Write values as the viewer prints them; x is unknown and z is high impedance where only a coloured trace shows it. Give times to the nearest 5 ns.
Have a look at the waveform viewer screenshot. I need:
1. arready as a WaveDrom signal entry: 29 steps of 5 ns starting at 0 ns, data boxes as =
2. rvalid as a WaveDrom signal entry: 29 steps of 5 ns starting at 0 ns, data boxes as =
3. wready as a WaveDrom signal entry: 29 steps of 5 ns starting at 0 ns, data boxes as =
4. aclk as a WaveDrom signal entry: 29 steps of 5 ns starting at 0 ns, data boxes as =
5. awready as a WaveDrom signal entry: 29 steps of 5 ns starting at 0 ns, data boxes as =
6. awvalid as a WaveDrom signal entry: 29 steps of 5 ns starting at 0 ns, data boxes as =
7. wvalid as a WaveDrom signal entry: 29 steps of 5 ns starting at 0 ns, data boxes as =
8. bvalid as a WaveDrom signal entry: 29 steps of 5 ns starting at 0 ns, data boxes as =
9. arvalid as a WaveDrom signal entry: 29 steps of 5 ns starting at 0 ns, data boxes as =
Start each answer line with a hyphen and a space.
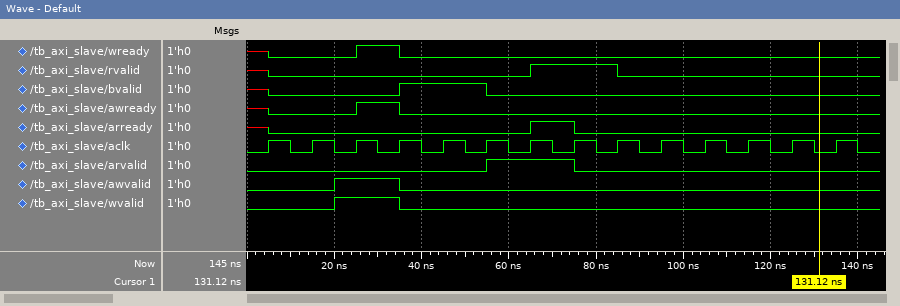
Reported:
- {name: 'arready', wave: 'x0...........1.0.............'}
- {name: 'rvalid', wave: 'x0...........1...0...........'}
- {name: 'wready', wave: 'x0...1.0.....................'}
- {name: 'aclk', wave: '01010101010101010101010101010'}
- {name: 'awready', wave: 'x0...1.0.....................'}
- {name: 'awvalid', wave: '0...1..0.....................'}
- {name: 'wvalid', wave: '0...1..0.....................'}
- {name: 'bvalid', wave: 'x0.....1...0.................'}
- {name: 'arvalid', wave: '0..........1...0.............'}
